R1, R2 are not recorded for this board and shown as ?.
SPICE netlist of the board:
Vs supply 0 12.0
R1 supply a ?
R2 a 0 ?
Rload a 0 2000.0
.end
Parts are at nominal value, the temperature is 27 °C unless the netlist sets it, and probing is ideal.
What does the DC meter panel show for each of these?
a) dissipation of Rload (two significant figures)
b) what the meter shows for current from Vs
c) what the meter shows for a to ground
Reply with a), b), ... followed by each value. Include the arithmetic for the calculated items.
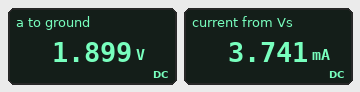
a) (1.899 V)^2 / 2 kΩ = 1.8 mW
b) 3.741 mA
c) 1.899 V
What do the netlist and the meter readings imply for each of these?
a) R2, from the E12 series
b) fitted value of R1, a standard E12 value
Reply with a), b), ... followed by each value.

a) 680 Ω
b) 2.7 kΩ
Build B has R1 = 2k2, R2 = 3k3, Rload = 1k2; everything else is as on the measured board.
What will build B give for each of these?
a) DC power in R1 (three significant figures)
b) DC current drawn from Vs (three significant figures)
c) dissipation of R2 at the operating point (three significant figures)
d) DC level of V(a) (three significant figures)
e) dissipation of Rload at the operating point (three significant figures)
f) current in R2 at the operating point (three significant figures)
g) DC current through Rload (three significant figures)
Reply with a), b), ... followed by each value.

a) 33.4 mW
b) 3.90 mA
c) 3.56 mW
d) 3.43 V
e) 9.80 mW
f) 1.04 mA
g) 2.86 mA
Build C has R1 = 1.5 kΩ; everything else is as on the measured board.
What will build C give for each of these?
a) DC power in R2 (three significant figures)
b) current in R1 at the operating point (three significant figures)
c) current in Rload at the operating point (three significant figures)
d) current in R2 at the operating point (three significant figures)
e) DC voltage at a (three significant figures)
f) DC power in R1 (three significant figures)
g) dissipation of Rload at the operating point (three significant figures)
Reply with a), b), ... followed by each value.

a) 13.5 mW
b) 5.98 mA
c) 1.52 mA
d) 4.46 mA
e) 3.03 V
f) 53.6 mW
g) 4.60 mW
